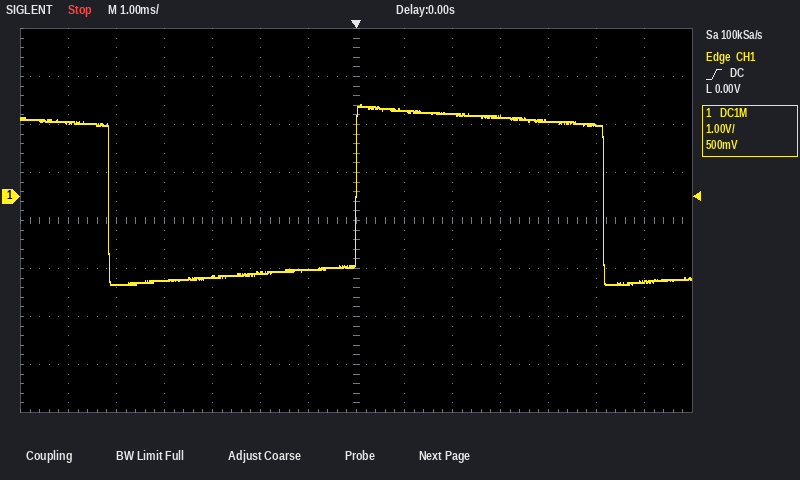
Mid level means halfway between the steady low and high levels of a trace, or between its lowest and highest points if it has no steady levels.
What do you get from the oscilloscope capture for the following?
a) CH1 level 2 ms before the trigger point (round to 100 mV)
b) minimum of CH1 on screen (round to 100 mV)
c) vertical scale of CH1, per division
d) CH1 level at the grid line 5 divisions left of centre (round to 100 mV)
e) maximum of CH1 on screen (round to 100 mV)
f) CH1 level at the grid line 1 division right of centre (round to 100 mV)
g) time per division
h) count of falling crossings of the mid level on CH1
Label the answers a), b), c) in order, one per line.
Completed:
a) -1.6 V
b) -1.8 V
c) 1 V
d) -1.8 V
e) 1.9 V
f) 1.8 V
g) 1 ms
h) 2
